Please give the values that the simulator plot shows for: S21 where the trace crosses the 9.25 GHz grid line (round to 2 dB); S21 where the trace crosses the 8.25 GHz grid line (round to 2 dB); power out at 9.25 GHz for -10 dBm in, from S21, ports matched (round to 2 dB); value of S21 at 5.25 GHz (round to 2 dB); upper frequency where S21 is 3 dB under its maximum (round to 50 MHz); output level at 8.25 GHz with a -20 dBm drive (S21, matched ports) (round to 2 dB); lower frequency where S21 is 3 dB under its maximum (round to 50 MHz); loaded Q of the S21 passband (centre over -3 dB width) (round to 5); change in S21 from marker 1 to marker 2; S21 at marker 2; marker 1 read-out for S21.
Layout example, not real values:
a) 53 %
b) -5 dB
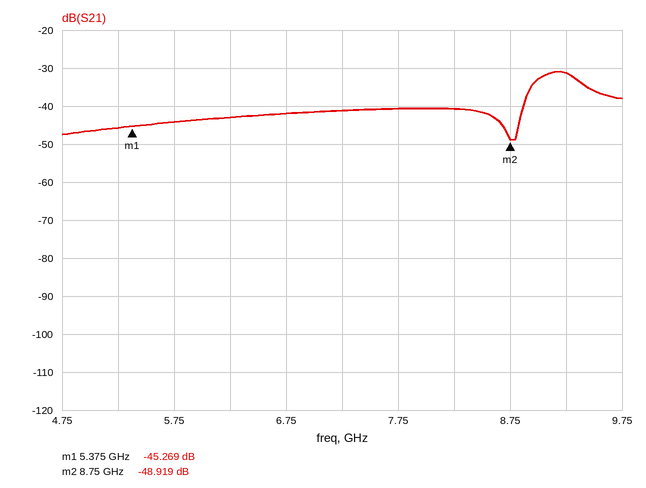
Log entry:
a) -32 dB
b) -40 dB
c) -42 dBm
d) -46 dB
e) 9.40 GHz
f) -60 dBm
g) 8.95 GHz
h) 20
i) -3.650 dB
j) -48.919 dB
k) -45.269 dB
